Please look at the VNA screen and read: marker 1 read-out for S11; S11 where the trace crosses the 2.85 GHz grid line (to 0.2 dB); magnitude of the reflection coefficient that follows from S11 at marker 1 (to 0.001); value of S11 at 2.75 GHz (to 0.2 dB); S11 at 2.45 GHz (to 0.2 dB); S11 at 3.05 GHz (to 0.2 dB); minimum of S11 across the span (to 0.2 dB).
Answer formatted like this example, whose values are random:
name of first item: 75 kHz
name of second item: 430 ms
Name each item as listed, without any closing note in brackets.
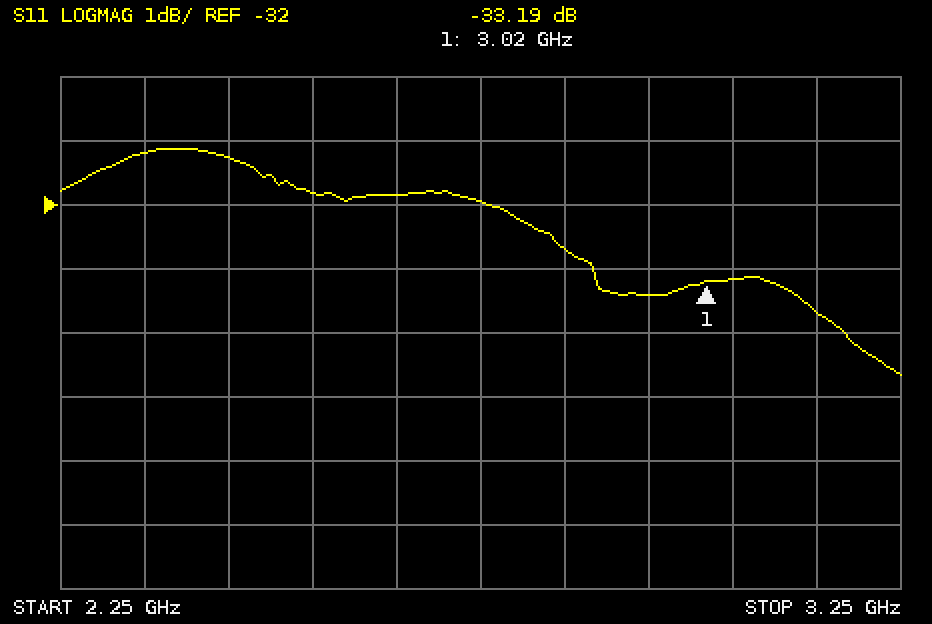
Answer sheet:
marker 1 read-out for S11: -33.19 dB
S11 where the trace crosses the 2.85 GHz grid line: -32.6 dB
magnitude of the reflection coefficient that follows from S11 at marker 1: 0.022
value of S11 at 2.75 GHz: -32.0 dB
S11 at 2.45 GHz: -31.2 dB
S11 at 3.05 GHz: -33.2 dB
minimum of S11 across the span: -34.6 dB
